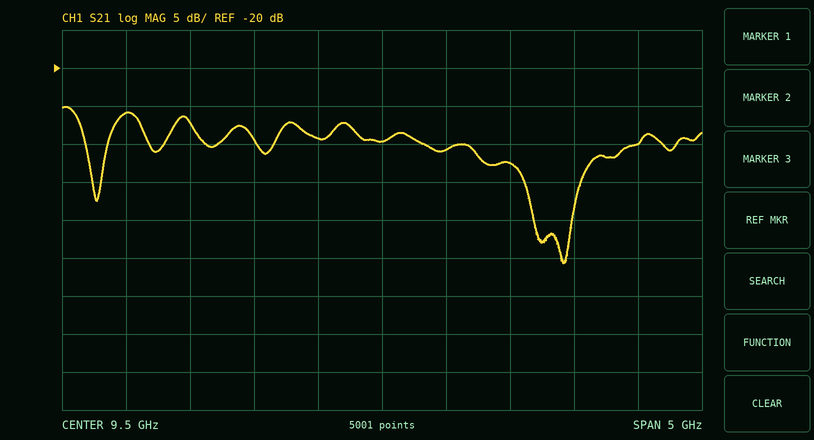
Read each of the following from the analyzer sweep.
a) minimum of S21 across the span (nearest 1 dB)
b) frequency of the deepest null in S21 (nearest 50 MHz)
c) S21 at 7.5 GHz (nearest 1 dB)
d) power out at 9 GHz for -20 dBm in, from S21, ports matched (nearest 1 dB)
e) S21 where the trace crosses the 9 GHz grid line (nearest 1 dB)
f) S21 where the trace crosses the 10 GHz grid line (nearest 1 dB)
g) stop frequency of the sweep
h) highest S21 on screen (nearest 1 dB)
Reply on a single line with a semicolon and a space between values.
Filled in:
-46 dB; 10.90 GHz; -26 dB; -49 dBm; -29 dB; -31 dB; 12 GHz; -25 dB
